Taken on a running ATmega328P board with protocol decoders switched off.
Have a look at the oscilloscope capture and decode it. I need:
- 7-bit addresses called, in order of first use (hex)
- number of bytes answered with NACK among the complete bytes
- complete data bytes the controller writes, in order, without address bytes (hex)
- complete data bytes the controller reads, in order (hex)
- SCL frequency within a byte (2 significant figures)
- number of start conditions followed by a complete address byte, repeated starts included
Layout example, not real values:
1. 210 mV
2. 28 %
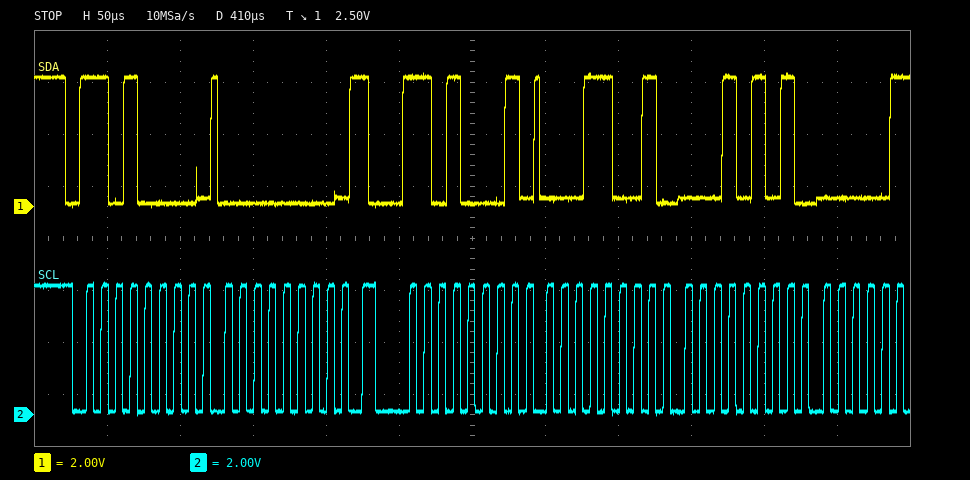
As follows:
1. 0x68
2. 0
3. 00
4. 19 15
5. 100 kHz
6. 2
